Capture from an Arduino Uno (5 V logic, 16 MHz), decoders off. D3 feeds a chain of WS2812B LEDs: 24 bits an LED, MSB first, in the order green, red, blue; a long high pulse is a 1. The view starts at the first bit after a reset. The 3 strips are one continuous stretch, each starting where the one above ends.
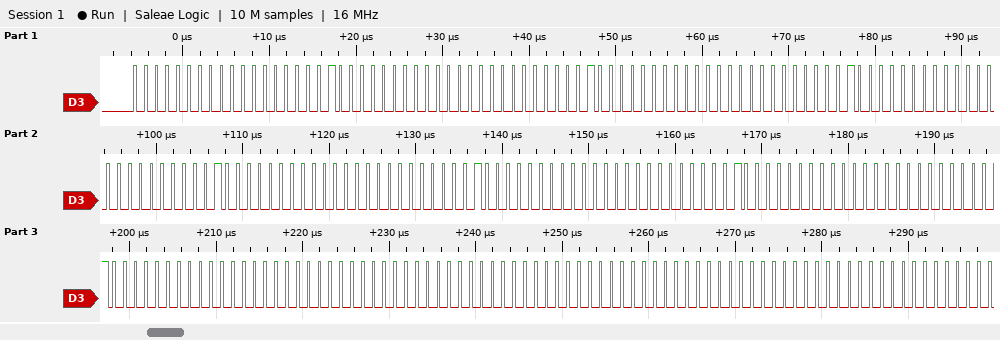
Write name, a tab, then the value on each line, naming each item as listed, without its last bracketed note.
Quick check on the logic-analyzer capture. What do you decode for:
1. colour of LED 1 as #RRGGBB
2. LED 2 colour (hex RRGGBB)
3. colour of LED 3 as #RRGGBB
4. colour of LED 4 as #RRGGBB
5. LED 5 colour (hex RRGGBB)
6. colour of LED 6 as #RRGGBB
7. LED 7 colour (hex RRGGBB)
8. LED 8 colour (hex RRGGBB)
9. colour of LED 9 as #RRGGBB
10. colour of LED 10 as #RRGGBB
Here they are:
colour of LED 1 as #RRGGBB	#000020
LED 2 colour	#000020
colour of LED 3 as #RRGGBB	#000020
colour of LED 4 as #RRGGBB	#000020
LED 5 colour	#000020
colour of LED 6 as #RRGGBB	#000020
LED 7 colour	#000020
LED 8 colour	#000000
colour of LED 9 as #RRGGBB	#000000
colour of LED 10 as #RRGGBB	#000000
